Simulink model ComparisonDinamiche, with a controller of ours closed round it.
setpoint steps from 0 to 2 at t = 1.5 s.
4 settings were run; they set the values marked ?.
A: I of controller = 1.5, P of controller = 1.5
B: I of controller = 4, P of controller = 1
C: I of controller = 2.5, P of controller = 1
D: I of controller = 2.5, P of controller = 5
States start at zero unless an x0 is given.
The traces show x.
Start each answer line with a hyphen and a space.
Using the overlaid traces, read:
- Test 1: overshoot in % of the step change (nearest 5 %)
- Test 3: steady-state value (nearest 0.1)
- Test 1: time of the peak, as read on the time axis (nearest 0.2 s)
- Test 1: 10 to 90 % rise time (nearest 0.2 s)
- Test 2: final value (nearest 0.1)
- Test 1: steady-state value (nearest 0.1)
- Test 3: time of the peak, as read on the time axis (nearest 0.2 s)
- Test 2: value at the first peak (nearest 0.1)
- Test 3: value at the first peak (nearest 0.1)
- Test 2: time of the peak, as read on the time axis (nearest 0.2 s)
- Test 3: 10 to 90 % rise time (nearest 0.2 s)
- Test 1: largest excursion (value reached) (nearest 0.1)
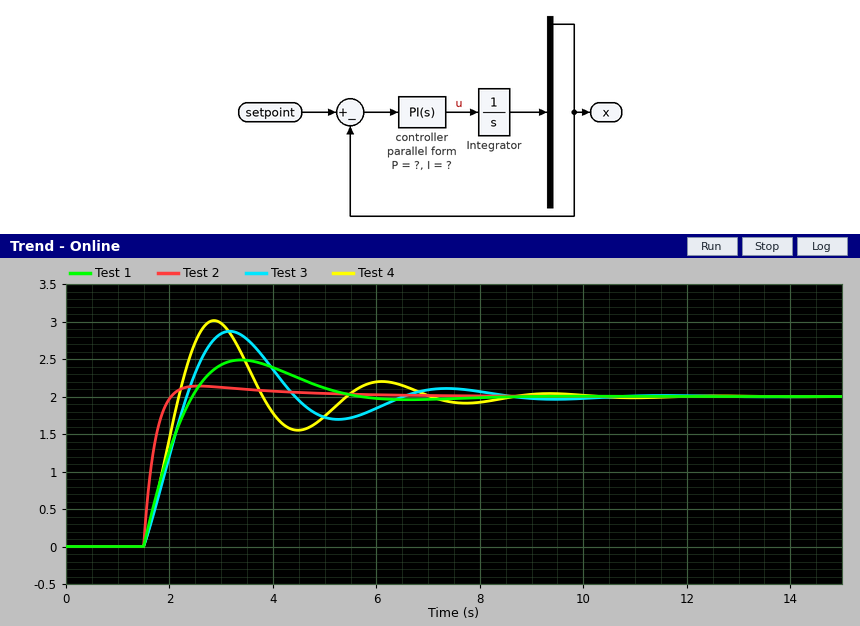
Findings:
- 25 %
- 2.0
- 3.4 s
- 0.8 s
- 2.0
- 2.0
- 3.2 s
- 2.1
- 2.9
- 2.6 s
- 0.6 s
- 2.5
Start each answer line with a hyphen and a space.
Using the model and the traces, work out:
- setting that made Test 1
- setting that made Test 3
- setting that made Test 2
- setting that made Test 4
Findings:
- A
- C
- D
- B
